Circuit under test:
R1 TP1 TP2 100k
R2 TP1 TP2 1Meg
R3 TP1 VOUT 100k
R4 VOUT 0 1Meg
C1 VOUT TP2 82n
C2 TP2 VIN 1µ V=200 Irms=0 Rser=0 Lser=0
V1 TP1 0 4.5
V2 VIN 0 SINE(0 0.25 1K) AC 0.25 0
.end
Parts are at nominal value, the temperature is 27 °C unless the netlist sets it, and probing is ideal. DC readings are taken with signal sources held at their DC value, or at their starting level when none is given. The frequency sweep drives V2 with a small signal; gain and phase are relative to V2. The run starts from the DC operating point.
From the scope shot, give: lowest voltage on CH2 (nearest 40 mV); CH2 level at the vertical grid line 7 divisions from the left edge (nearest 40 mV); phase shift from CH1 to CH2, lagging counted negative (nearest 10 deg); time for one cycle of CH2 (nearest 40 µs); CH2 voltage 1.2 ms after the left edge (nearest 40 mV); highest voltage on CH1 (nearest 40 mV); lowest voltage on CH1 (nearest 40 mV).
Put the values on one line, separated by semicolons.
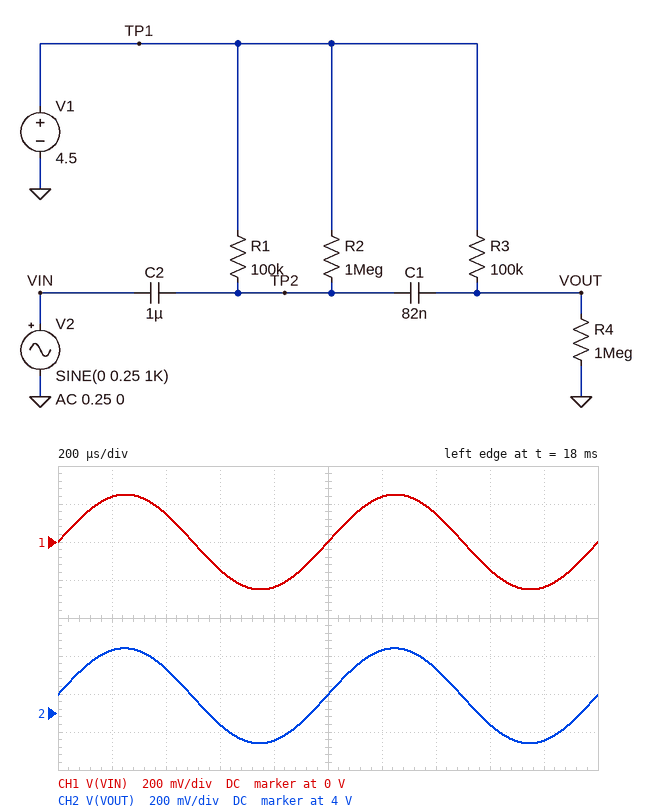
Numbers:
3.84 V; 4.24 V; 0 deg; 1.00 ms; 4.32 V; 240 mV; -240 mV
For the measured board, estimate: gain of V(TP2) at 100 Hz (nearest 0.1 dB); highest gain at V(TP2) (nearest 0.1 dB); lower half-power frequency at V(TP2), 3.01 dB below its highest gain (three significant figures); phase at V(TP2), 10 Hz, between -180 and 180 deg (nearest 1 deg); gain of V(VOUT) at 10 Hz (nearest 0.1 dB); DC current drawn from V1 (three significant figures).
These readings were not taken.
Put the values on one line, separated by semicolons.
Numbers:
0 dB; 0 dB; 1.94 Hz; 11 deg; -8.2 dB; 4.09 µA
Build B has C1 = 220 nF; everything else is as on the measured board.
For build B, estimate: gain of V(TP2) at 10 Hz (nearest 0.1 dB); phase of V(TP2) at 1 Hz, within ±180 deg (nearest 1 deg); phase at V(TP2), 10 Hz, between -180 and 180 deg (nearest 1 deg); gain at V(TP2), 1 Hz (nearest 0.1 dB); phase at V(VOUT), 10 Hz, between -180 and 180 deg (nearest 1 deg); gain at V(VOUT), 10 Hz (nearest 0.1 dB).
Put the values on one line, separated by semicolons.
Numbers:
-1.0 dB; 56 deg; 15 deg; -6.7 dB; 53 deg; -3.1 dB
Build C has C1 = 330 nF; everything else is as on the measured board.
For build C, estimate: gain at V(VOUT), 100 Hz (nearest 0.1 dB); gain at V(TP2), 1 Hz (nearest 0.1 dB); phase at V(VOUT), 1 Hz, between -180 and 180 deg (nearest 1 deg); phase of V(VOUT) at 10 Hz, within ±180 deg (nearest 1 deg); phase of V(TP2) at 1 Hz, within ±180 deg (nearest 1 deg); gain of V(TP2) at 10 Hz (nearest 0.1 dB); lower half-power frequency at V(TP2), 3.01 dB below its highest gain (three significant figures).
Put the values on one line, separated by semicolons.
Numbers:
0 dB; -7.0 dB; 133 deg; 44 deg; 54 deg; -1.0 dB; 3.28 Hz
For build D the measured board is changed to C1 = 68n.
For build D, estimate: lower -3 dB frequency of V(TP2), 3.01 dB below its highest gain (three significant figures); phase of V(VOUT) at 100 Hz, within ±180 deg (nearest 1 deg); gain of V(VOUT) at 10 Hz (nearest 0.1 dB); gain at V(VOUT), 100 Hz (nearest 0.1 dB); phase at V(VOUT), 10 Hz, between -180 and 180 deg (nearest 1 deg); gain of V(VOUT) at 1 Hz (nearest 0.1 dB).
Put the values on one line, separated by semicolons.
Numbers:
1.90 Hz; 16 deg; -9.5 dB; -0.3 dB; 79 deg; -34.5 dB
